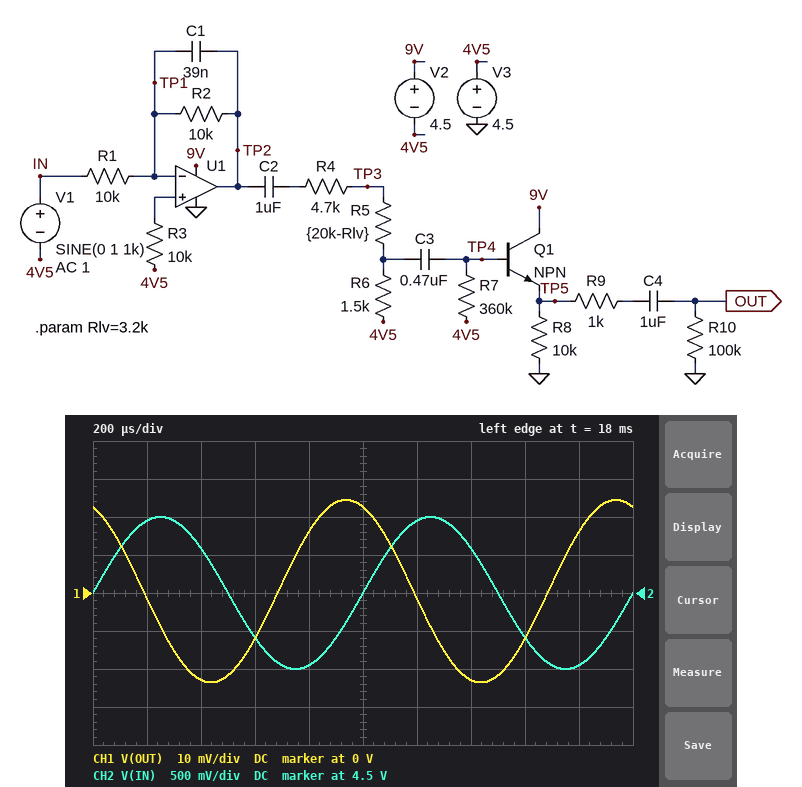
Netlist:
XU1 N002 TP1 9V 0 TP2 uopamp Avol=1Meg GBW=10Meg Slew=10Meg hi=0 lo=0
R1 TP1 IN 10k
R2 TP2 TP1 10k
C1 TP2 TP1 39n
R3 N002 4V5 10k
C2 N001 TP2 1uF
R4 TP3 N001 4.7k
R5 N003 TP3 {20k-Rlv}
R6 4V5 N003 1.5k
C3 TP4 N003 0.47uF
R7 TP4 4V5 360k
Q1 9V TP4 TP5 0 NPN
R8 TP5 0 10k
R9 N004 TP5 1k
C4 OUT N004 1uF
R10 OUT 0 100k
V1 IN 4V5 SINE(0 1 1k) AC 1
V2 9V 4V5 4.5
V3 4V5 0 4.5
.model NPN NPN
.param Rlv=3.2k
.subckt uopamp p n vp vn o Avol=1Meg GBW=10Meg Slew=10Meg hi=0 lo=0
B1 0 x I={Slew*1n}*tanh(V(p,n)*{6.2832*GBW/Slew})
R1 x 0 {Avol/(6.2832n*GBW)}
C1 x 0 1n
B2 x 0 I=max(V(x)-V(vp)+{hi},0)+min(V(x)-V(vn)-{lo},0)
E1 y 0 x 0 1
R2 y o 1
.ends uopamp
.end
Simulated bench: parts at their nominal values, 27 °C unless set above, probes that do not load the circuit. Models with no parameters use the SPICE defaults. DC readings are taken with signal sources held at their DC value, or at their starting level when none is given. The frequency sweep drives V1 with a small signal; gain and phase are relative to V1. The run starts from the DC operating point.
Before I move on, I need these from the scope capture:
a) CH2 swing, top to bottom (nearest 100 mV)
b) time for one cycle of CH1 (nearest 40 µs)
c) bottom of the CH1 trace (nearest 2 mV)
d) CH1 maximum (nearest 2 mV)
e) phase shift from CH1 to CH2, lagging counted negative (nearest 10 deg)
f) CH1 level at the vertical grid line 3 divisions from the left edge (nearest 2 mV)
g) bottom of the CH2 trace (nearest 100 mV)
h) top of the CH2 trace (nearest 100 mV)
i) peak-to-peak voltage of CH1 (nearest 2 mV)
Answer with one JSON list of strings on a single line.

["2.0 V", "1.00 ms", "-24 mV", "24 mV", "-110 deg", "-12 mV", "3.5 V", "5.5 V", "48 mV"]
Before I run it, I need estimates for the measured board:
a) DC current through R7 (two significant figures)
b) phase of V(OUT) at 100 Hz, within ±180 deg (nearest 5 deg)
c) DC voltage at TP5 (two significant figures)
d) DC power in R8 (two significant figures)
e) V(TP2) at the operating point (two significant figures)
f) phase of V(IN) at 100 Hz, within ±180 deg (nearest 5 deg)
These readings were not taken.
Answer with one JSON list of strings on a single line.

["2.7 µA", "170 deg", "2.8 V", "770 µW", "4.5 V", "0 deg"]
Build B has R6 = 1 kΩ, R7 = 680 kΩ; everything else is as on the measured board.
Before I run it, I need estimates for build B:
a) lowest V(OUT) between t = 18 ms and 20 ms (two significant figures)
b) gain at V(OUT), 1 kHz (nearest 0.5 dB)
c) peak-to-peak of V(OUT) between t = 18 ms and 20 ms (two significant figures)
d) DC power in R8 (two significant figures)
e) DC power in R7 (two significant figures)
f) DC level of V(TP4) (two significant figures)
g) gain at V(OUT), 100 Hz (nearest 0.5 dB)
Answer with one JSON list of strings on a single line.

["-16 mV", "-35.5 dB", "33 mV", "510 µW", "3.4 µW", "3.0 V", "-27.5 dB"]
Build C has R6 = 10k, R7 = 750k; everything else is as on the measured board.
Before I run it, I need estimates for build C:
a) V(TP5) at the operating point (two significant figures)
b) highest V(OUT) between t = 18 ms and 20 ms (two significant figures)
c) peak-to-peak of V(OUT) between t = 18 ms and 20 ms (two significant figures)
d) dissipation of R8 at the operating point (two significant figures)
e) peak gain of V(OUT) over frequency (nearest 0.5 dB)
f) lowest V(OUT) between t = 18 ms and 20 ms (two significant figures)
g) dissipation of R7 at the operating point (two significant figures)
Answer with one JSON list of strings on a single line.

["2.2 V", "120 mV", "230 mV", "470 µW", "-10.5 dB", "-110 mV", "3.4 µW"]
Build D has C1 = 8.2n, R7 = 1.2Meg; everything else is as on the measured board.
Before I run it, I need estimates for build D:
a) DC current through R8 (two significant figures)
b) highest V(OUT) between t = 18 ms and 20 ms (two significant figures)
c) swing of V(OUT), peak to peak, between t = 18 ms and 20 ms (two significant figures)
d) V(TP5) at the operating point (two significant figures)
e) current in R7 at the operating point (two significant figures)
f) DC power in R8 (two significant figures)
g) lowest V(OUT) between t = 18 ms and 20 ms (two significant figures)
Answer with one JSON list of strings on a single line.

["170 µA", "57 mV", "110 mV", "1.7 V", "1.7 µA", "300 µW", "-56 mV"]
